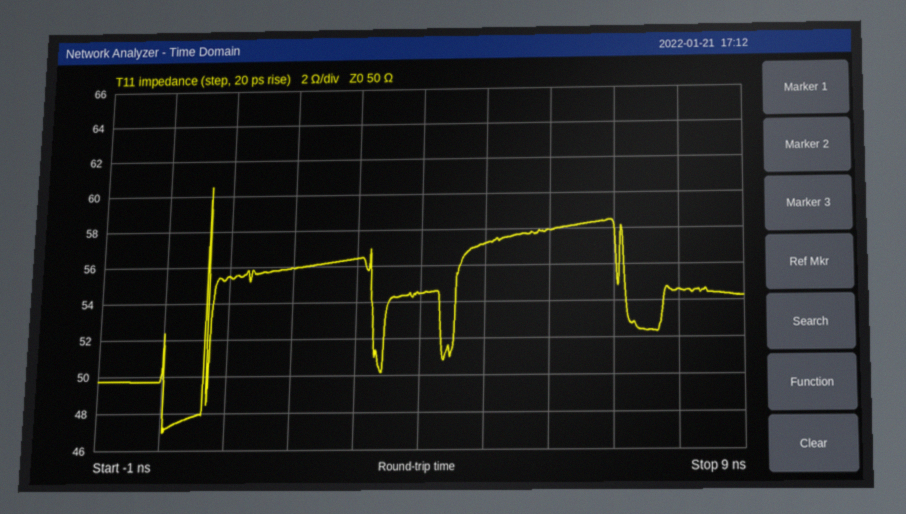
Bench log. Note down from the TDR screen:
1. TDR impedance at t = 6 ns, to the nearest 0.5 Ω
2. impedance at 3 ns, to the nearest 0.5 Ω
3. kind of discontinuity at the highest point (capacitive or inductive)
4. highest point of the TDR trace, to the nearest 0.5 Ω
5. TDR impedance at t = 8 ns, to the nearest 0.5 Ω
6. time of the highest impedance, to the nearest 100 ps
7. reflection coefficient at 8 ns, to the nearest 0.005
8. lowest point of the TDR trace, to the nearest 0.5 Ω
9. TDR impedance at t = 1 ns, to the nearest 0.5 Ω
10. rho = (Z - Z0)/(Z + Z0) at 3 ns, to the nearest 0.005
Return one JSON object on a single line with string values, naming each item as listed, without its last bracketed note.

{"TDR impedance at t = 6 ns, to the nearest 0.5 Ω": "58.0 Ω", "impedance at 3 ns, to the nearest 0.5 Ω": "56.5 Ω", "kind of discontinuity at the highest point": "inductive", "highest point of the TDR trace, to the nearest 0.5 Ω": "60.5 Ω", "TDR impedance at t = 8 ns, to the nearest 0.5 Ω": "54.5 Ω", "time of the highest impedance, to the nearest 100 ps": "700 ps", "reflection coefficient at 8 ns, to the nearest 0.005": "+0.045", "lowest point of the TDR trace, to the nearest 0.5 Ω": "47.0 Ω", "TDR impedance at t = 1 ns, to the nearest 0.5 Ω": "55.5 Ω", "rho = (Z - Z0)/(Z + Z0) at 3 ns, to the nearest 0.005": "+0.060"}
